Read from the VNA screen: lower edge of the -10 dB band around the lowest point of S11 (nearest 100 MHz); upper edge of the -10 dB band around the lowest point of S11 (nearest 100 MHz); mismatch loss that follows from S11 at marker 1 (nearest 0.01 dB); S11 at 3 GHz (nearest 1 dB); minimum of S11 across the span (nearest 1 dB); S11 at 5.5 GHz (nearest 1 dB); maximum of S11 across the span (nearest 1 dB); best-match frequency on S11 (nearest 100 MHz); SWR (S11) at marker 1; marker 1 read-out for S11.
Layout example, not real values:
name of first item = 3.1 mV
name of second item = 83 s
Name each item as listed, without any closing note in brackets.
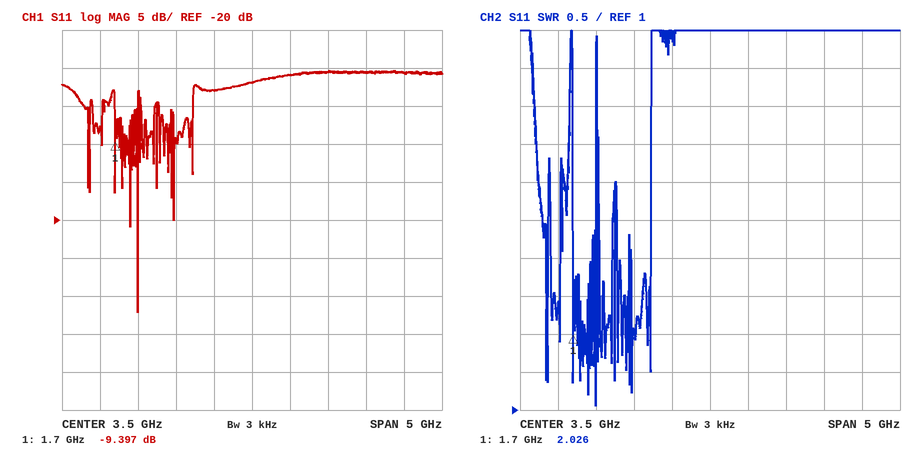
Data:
lower edge of the -10 dB band around the lowest point of S11 = 2.0 GHz
upper edge of the -10 dB band around the lowest point of S11 = 2.0 GHz
mismatch loss that follows from S11 at marker 1 = 0.53 dB
S11 at 3 GHz = -3 dB
minimum of S11 across the span = -32 dB
S11 at 5.5 GHz = -1 dB
maximum of S11 across the span = 0 dB
best-match frequency on S11 = 2.0 GHz
SWR (S11) at marker 1 = 2.026
marker 1 read-out for S11 = -9.397 dB
